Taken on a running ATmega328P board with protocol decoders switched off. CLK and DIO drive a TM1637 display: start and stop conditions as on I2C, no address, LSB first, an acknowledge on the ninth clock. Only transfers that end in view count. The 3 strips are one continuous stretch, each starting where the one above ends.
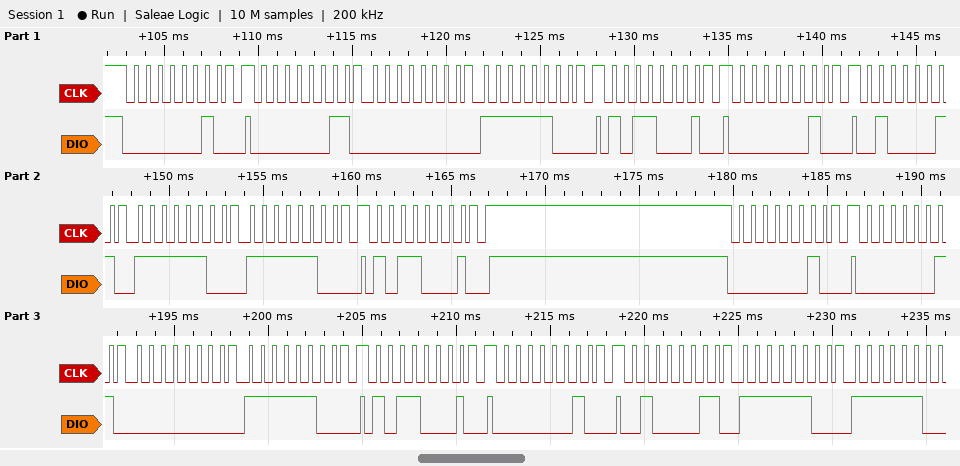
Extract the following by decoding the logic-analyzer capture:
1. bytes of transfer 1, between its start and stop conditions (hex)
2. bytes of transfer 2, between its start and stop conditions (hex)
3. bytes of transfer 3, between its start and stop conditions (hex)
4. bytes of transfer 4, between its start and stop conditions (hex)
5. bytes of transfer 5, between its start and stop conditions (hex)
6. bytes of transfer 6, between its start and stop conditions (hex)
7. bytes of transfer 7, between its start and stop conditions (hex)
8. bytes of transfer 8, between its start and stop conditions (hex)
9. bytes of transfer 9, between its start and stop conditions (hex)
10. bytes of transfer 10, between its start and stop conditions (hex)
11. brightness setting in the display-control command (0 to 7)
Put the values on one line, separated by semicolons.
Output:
40; C0 00 3F; 8D; 40; C2 3F 3F; 8D; 40; C0 00 3F; 8D; 40; 5
